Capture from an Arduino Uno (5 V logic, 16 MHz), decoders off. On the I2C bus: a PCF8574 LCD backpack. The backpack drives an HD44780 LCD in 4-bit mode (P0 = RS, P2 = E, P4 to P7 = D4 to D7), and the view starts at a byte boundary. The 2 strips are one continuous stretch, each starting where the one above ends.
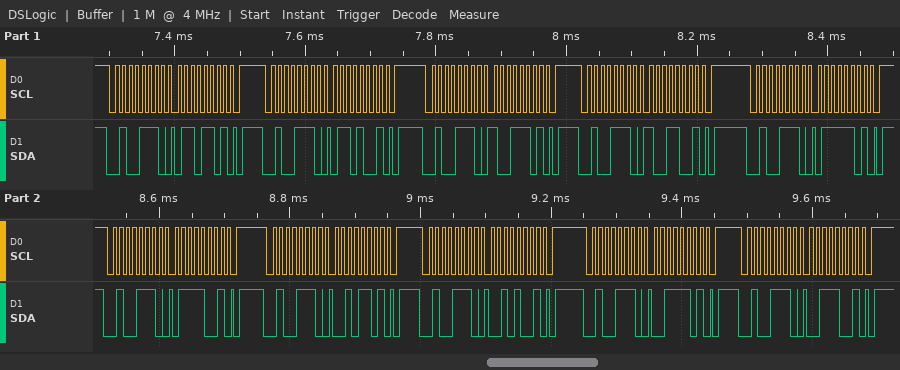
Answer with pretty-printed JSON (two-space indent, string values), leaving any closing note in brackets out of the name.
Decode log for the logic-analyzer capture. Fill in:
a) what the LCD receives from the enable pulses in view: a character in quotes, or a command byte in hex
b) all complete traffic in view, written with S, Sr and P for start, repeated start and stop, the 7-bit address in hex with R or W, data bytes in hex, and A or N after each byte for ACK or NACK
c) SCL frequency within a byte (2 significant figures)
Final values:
{
  "what the LCD receives from the enable pulses in view: a character in quotes, or a command byte in hex": "'i' 'r'",
  "all complete traffic in view, written with S, Sr and P for start, repeated start and stop, the 7-bit address in hex with R or W, data bytes in hex, and A or N after each byte for ACK or NACK": "S 27W A 6D A P S 27W A 69 A P S 27W A 9D A P S 27W A 99 A P S 27W A 7D A P S 27W A 79 A P S 27W A 2D A P S 27W A 29 A P S 27W A 3D A P S 27W A 39 A P",
  "SCL frequency within a byte": "100 kHz"
}
